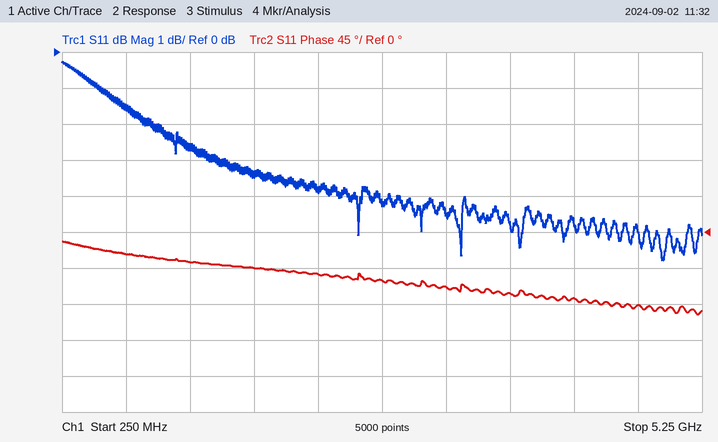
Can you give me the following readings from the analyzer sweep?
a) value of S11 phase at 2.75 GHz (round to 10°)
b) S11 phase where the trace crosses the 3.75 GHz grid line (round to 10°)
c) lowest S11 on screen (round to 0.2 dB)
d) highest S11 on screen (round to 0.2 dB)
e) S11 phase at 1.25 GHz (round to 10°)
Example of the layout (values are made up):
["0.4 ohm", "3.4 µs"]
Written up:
["-60°", "-80°", "-5.8 dB", "-0.2 dB", "-40°"]
